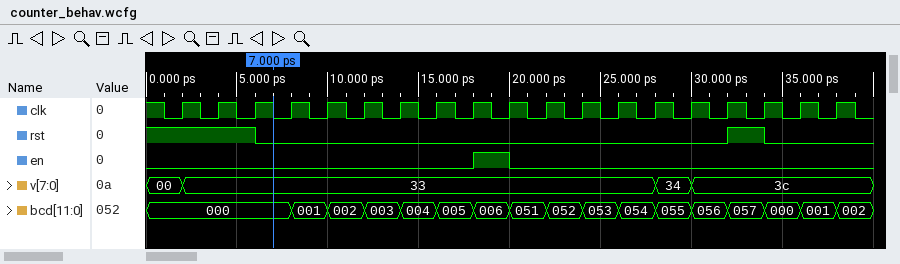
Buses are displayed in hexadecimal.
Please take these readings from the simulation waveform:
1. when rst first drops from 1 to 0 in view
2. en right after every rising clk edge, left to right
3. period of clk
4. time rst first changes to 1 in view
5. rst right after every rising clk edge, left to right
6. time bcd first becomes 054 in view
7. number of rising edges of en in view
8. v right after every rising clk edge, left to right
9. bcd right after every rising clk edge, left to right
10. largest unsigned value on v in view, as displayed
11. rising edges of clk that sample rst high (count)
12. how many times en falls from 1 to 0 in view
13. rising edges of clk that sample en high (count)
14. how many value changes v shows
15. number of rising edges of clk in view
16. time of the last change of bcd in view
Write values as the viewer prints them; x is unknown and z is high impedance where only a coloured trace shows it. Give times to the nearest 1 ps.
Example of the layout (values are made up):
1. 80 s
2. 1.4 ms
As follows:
1. 6 ps
2. 0 0 0 0 0 0 0 0 1 0 0 0 0 0 0 0 0 0 0
3. 2 ps
4. 32 ps
5. 1 1 0 0 0 0 0 0 0 0 0 0 0 0 0 1 0 0 0
6. 26 ps
7. 1
8. 33, 33, 33, 33, 33, 33, 33, 33, 33, 33, 33, 33, 33, 34, 3c, 3c, 3c, 3c, 3c
9. 000, 000, 000, 001, 002, 003, 004, 005, 006, 051, 052, 053, 054, 055, 056, 057, 000, 001, 002
10. 3c
11. 4
12. 1
13. 1
14. 3
15. 19
16. 38 ps
